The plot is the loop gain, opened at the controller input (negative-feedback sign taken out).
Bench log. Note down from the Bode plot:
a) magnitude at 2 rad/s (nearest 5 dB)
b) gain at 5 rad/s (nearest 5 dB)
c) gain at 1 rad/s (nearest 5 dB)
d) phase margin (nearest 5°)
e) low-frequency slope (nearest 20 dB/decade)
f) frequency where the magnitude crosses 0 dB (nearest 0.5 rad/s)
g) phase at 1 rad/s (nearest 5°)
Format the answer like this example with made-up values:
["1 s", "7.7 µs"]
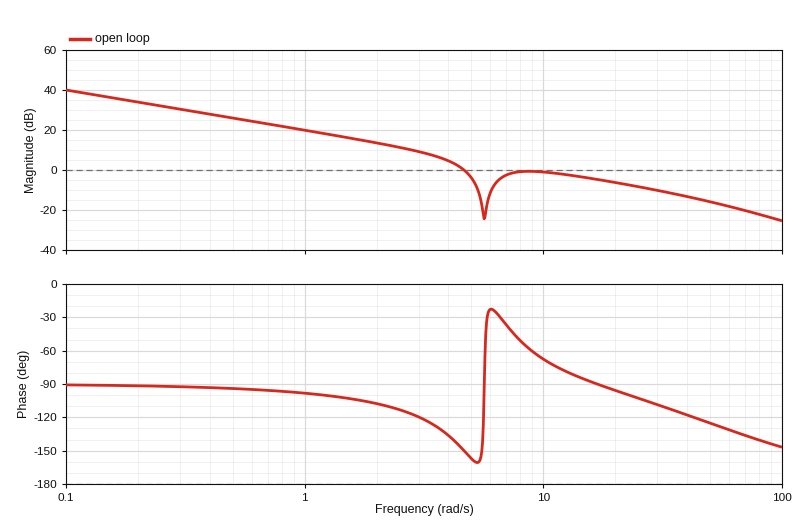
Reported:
["15 dB", "-5 dB", "20 dB", "30°", "-20 dB/decade", "4.5 rad/s", "-100°"]
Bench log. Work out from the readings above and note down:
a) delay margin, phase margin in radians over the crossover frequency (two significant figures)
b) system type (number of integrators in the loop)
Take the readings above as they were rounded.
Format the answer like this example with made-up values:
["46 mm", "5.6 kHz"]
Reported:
["0.12 s", "1"]
